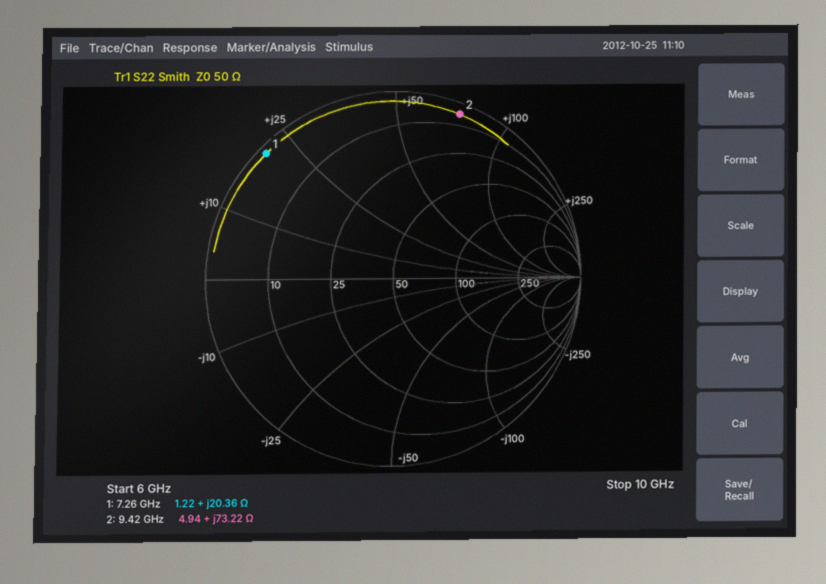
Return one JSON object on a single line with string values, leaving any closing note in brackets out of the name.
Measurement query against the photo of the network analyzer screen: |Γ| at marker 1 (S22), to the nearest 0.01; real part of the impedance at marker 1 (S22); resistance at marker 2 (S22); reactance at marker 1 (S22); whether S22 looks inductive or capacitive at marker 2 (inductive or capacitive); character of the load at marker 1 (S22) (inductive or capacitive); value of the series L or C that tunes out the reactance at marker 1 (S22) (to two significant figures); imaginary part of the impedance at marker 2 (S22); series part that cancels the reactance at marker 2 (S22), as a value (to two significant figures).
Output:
{"|Γ| at marker 1 (S22), to the nearest 0.01": "0.96", "real part of the impedance at marker 1": "1.22 Ω", "resistance at marker 2": "4.94 Ω", "reactance at marker 1": "+20.36 Ω", "whether S22 looks inductive or capacitive at marker 2": "inductive", "character of the load at marker 1 (S22)": "inductive", "value of the series L or C that tunes out the reactance at marker 1 (S22)": "1.1 pF", "imaginary part of the impedance at marker 2": "+73.22 Ω", "series part that cancels the reactance at marker 2 (S22), as a value": "230 fF"}
